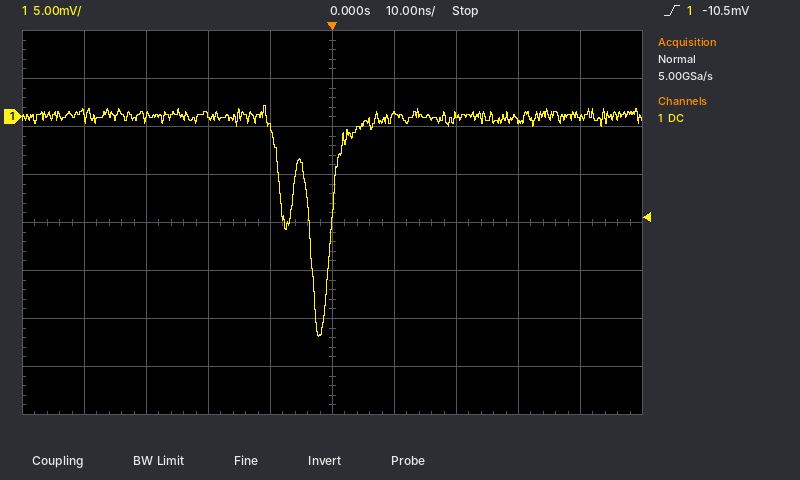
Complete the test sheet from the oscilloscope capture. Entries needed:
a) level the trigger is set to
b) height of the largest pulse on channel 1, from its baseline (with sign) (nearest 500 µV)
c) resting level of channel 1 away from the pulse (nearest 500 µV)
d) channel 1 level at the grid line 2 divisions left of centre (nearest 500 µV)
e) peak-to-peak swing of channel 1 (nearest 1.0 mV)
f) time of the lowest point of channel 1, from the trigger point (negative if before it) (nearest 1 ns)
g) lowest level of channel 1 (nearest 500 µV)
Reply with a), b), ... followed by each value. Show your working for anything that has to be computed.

a) -10.5 mV
b) -23.0 mV − (0.0 mV) = -23.0 mV
c) 0.0 mV
d) 0.0 mV
e) 24.0 mV
f) -2 ns
g) -23.0 mV
